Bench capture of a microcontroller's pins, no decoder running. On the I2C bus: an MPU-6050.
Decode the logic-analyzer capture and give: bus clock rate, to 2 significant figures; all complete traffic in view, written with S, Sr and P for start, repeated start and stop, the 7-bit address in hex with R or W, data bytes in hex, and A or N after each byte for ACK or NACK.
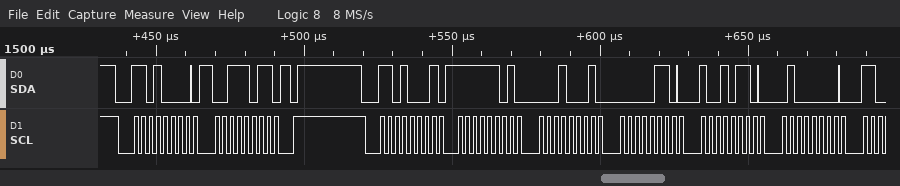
400 kHz
S 68W A 3B A P S 68R A FD A 11 A 06 A 96 A 40 A
